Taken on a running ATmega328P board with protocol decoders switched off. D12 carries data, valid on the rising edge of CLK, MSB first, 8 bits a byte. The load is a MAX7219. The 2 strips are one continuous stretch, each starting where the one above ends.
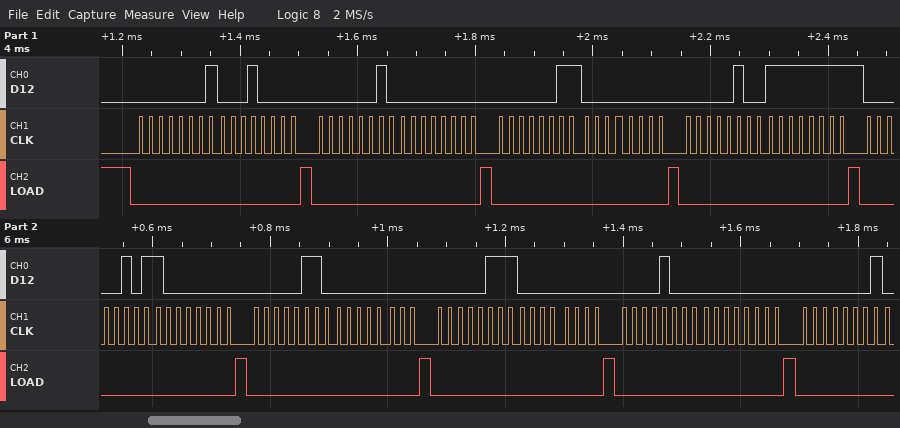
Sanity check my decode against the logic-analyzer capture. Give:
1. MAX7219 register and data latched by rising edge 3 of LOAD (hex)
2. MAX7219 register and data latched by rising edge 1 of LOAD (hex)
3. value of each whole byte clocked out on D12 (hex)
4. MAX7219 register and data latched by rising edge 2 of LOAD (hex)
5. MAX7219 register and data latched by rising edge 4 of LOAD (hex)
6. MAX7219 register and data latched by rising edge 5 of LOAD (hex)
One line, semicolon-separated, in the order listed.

register 0x3, data 0x00; register 0x1, data 0x10; 01 10 02 00 03 00 04 FF 05 80 06 00 07 00 08 00 01; register 0x2, data 0x00; register 0x4, data 0xFF; register 0x5, data 0x80
